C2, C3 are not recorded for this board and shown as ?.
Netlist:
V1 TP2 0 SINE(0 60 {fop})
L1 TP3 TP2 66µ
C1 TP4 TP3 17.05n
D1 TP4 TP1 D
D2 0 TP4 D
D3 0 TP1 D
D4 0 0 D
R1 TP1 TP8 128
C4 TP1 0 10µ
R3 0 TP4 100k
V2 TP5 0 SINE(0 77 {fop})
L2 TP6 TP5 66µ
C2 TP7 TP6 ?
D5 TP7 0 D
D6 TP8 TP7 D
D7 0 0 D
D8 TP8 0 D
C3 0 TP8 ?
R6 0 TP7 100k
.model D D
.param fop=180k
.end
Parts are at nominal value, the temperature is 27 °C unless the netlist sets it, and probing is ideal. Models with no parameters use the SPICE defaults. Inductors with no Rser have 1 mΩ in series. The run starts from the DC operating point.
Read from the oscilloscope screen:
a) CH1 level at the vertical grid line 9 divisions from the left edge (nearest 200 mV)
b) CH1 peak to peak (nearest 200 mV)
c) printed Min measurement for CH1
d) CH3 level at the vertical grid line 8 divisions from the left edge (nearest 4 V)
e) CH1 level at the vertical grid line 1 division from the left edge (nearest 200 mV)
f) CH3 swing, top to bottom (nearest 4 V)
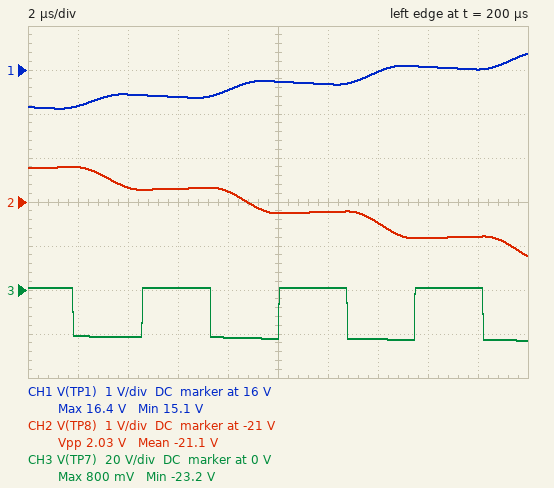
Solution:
16.0 V
1.2 V
15.1 V
0 V
15.2 V
24 V
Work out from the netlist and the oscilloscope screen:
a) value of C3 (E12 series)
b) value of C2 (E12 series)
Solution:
18 µF
10 nF
